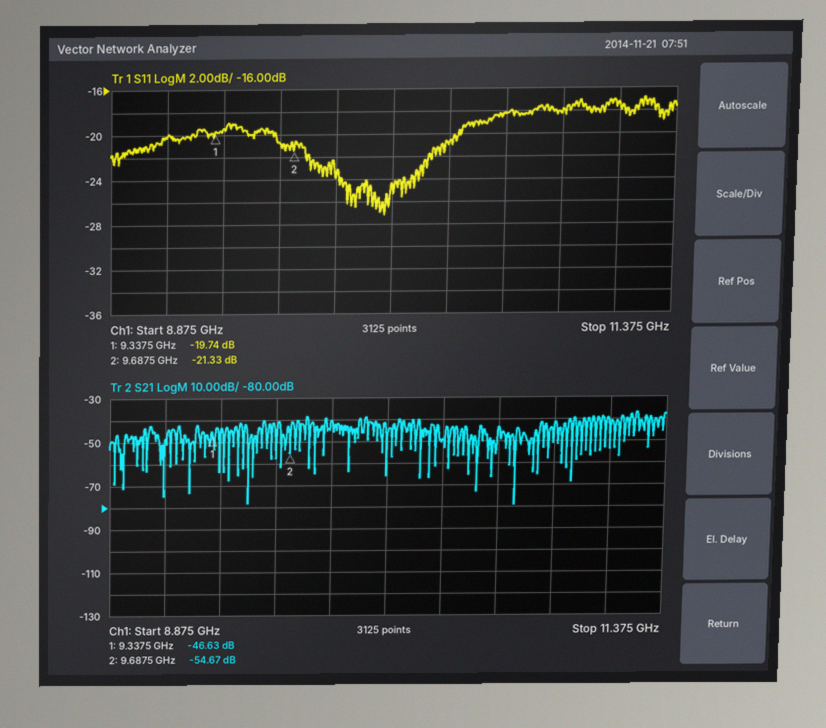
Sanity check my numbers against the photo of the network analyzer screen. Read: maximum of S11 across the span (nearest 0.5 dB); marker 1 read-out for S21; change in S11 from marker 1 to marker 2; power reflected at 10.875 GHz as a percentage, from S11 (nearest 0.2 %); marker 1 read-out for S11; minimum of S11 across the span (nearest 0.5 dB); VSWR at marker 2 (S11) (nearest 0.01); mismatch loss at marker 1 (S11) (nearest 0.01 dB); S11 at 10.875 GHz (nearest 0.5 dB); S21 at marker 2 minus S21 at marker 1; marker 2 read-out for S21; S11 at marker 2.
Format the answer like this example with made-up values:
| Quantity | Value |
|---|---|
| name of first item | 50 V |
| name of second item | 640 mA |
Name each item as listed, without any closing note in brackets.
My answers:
| Quantity | Value |
|---|---|
| maximum of S11 across the span | -17.0 dB |
| marker 1 read-out for S21 | -46.63 dB |
| change in S11 from marker 1 to marker 2 | -1.59 dB |
| power reflected at 10.875 GHz as a percentage, from S11 | 1.6 % |
| marker 1 read-out for S11 | -19.74 dB |
| minimum of S11 across the span | -27.0 dB |
| VSWR at marker 2 (S11) | 1.19 |
| mismatch loss at marker 1 (S11) | 0.05 dB |
| S11 at 10.875 GHz | -18.0 dB |
| S21 at marker 2 minus S21 at marker 1 | -8.04 dB |
| marker 2 read-out for S21 | -54.67 dB |
| S11 at marker 2 | -21.33 dB |
